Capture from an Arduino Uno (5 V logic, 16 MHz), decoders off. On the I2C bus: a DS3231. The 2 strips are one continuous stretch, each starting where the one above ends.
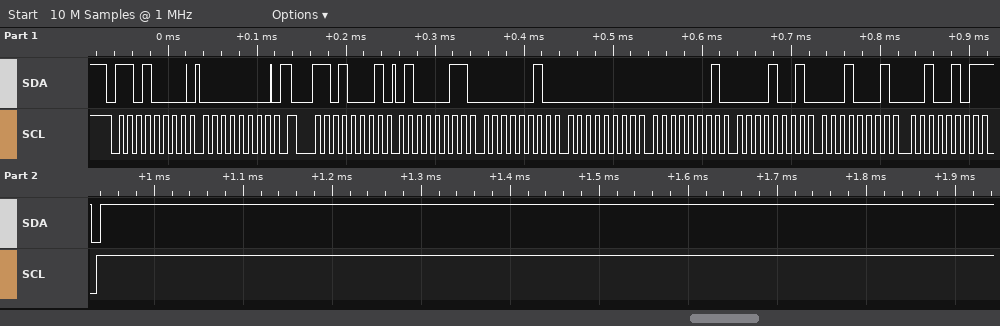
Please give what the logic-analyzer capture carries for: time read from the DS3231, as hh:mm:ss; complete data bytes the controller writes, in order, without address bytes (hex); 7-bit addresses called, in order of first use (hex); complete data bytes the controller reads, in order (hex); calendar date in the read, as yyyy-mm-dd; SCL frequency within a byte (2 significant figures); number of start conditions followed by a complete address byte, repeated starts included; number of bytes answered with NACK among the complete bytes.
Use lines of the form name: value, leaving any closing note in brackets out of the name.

time read from the DS3231, as hh:mm:ss: 00:02:43
complete data bytes the controller writes, in order, without address bytes: 00
7-bit addresses called, in order of first use: 0x68
complete data bytes the controller reads, in order: 43 02 00 01 09 11 25
calendar date in the read, as yyyy-mm-dd: 2025-11-09
SCL frequency within a byte: 100 kHz
number of start conditions followed by a complete address byte, repeated starts included: 2
number of bytes answered with NACK among the complete bytes: 1
